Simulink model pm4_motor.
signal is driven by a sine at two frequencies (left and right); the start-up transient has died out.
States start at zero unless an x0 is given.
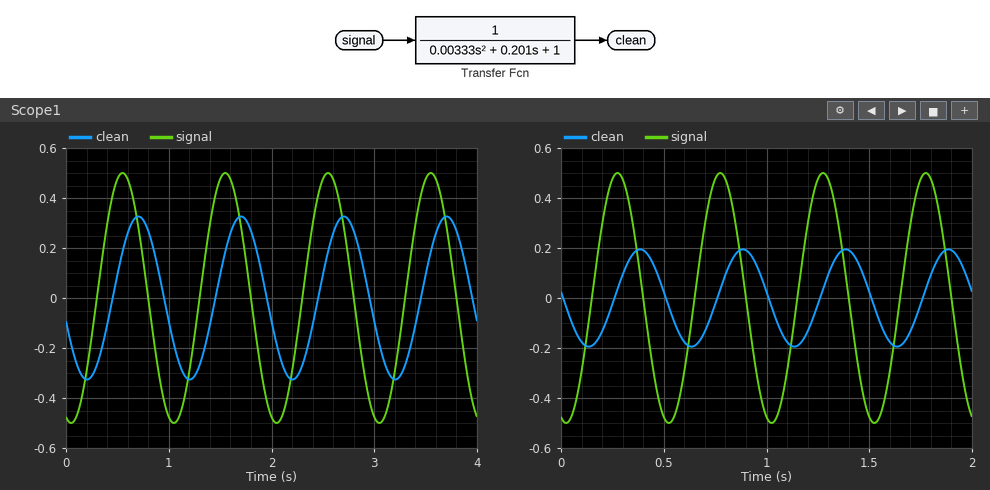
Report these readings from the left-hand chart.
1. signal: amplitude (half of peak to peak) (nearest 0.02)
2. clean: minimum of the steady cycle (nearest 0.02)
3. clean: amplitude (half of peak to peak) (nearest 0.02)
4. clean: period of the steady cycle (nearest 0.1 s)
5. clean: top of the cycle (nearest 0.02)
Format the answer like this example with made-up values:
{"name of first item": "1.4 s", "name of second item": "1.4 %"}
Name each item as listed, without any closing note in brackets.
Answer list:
{"signal: amplitude (half of peak to peak)": "0.50", "clean: minimum of the steady cycle": "-0.32", "clean: amplitude (half of peak to peak)": "0.32", "clean: period of the steady cycle": "1.0 s", "clean: top of the cycle": "0.32"}
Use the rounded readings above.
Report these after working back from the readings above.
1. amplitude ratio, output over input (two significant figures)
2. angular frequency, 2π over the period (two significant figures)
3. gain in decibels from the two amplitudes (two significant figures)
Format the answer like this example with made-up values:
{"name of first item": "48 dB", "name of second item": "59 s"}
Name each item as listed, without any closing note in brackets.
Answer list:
{"amplitude ratio, output over input": "0.64", "angular frequency, 2π over the period": "6.3 rad/s", "gain in decibels from the two amplitudes": "-3.9 dB"}
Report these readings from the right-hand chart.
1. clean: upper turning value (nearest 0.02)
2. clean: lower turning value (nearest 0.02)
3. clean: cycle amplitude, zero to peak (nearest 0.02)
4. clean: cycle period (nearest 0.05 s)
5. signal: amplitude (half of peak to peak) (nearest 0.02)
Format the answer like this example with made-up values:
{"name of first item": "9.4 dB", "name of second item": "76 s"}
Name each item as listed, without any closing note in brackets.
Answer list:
{"clean: upper turning value": "0.20", "clean: lower turning value": "-0.20", "clean: cycle amplitude, zero to peak": "0.20", "clean: cycle period": "0.50 s", "signal: amplitude (half of peak to peak)": "0.50"}
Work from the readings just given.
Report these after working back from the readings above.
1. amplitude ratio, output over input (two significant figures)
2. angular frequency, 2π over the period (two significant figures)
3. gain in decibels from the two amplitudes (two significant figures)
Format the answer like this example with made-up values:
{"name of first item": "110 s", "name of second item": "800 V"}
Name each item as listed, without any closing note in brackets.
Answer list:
{"amplitude ratio, output over input": "0.40", "angular frequency, 2π over the period": "13 rad/s", "gain in decibels from the two amplitudes": "-8.0 dB"}
